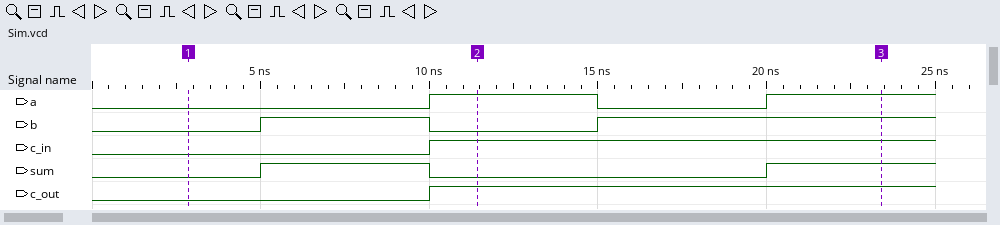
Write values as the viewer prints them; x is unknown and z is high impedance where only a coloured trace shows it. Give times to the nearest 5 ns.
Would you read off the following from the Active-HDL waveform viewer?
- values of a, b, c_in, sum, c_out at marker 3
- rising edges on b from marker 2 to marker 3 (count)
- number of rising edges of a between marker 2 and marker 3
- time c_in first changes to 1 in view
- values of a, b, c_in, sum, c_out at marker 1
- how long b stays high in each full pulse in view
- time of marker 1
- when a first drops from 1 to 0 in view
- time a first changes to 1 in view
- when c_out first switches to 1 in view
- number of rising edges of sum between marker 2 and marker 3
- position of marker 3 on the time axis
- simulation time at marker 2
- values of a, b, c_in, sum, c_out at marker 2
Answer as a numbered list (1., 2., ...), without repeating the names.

1. a=1, b=1, c_in=1, sum=1, c_out=1
2. 1
3. 1
4. 10 ns
5. a=0, b=0, c_in=0, sum=0, c_out=0
6. 5 ns
7. 5 ns
8. 15 ns
9. 10 ns
10. 10 ns
11. 1
12. 25 ns
13. 10 ns
14. a=1, b=0, c_in=1, sum=0, c_out=1
